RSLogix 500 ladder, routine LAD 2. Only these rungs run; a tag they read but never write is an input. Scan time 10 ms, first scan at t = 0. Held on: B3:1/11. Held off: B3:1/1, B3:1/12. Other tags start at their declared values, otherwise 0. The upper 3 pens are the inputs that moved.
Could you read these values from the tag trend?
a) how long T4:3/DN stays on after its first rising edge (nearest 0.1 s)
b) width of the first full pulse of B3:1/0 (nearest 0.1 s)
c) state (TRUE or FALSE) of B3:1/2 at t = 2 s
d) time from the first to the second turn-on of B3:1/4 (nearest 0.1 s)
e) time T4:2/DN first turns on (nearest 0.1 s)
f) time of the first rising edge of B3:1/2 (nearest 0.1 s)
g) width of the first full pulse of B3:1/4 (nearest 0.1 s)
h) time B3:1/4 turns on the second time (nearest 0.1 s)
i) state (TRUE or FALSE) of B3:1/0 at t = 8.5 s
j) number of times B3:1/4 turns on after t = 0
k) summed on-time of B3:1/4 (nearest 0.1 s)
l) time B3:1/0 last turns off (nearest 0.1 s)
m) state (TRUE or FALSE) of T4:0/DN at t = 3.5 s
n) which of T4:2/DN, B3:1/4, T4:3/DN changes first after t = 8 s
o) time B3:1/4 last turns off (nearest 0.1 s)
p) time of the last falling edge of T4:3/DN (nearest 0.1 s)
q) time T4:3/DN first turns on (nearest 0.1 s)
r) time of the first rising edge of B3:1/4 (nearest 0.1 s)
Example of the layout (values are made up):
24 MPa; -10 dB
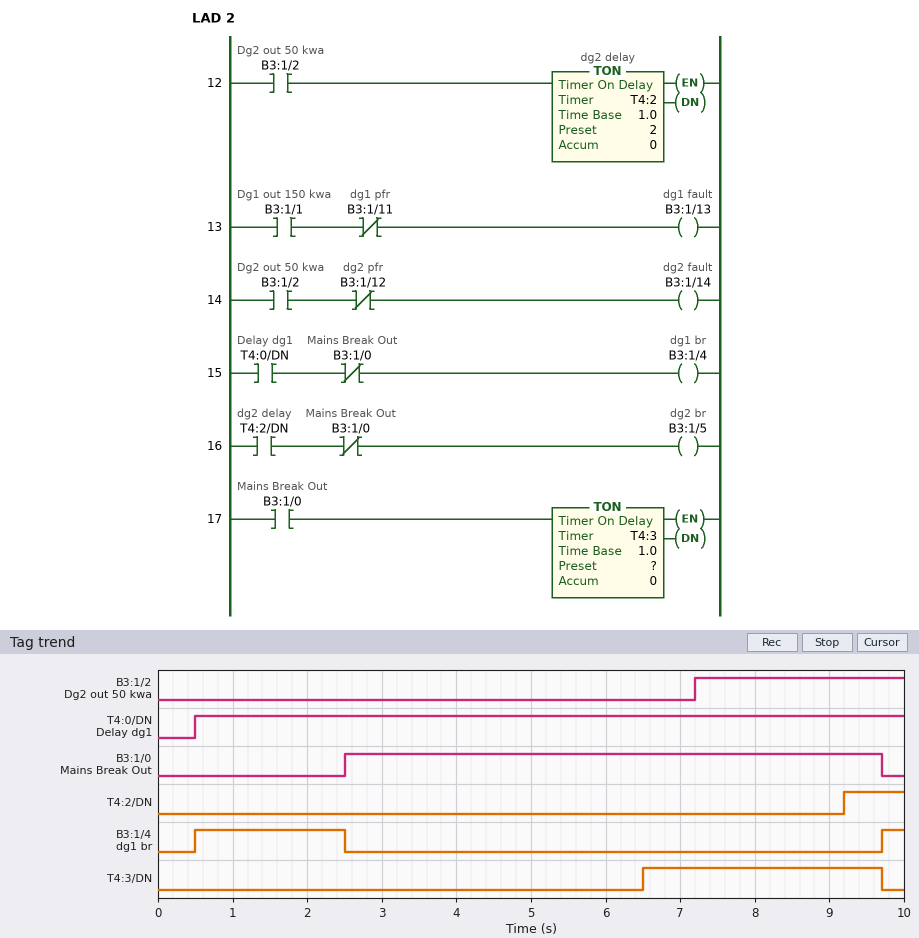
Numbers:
3.2 s; 7.2 s; FALSE; 9.2 s; 9.2 s; 7.2 s; 2.0 s; 9.7 s; TRUE; 2; 2.3 s; 9.7 s; TRUE; T4:2/DN; 2.5 s; 9.7 s; 6.5 s; 0.5 s
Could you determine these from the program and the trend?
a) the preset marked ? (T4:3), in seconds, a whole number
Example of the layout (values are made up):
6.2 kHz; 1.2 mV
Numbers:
4 s
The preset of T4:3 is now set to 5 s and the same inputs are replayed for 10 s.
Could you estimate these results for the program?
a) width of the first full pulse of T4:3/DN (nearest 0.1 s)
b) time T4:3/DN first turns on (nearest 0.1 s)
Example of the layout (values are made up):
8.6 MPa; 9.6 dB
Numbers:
2.2 s; 7.5 s
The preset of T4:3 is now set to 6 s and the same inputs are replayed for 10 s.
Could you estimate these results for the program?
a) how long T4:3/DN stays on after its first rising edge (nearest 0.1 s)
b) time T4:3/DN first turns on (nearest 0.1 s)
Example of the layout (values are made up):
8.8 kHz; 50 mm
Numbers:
1.2 s; 8.5 s
